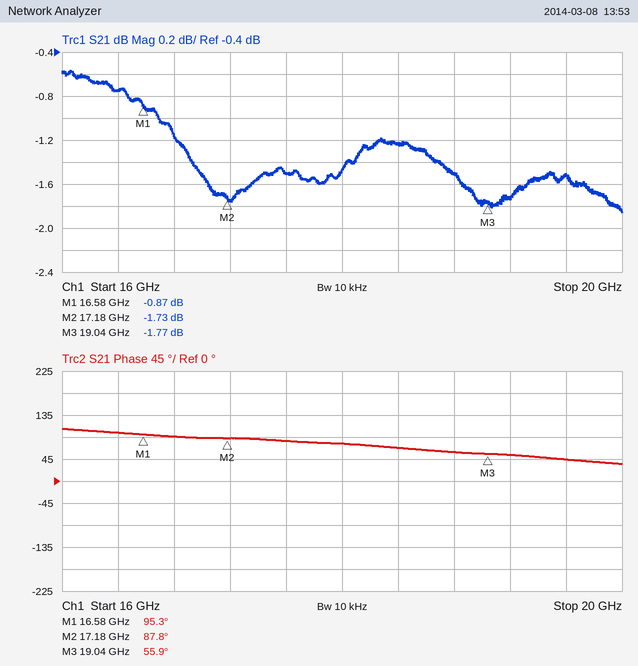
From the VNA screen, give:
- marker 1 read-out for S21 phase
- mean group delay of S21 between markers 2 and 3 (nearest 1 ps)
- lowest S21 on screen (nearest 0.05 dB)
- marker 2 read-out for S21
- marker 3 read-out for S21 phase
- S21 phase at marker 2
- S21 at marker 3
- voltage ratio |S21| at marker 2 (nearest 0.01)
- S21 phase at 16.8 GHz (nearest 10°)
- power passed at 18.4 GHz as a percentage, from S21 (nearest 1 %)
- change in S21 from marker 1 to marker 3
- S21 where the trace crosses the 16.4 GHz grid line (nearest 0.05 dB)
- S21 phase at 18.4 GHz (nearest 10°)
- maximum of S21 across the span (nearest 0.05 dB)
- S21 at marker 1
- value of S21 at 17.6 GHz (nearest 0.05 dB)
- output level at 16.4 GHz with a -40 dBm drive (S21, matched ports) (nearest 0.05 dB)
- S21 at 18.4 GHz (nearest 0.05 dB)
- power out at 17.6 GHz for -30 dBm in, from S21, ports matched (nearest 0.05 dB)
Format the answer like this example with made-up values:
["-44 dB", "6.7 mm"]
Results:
["95.3°", "48 ps", "-1.85 dB", "-1.73 dB", "55.9°", "87.8°", "-1.77 dB", "0.82", "90°", "75 %", "-0.90 dB", "-0.75 dB", "70°", "-0.55 dB", "-0.87 dB", "-1.50 dB", "-40.75 dBm", "-1.25 dB", "-31.50 dBm"]
